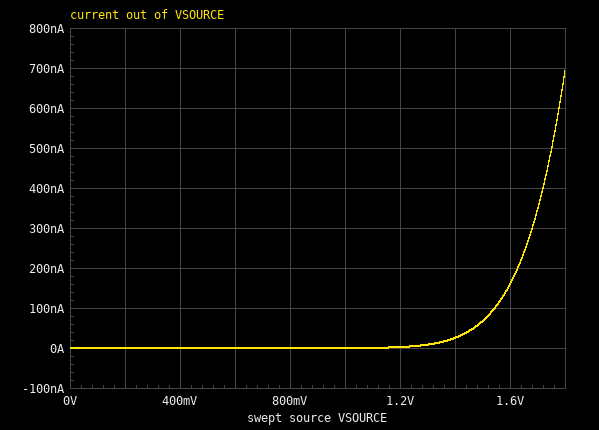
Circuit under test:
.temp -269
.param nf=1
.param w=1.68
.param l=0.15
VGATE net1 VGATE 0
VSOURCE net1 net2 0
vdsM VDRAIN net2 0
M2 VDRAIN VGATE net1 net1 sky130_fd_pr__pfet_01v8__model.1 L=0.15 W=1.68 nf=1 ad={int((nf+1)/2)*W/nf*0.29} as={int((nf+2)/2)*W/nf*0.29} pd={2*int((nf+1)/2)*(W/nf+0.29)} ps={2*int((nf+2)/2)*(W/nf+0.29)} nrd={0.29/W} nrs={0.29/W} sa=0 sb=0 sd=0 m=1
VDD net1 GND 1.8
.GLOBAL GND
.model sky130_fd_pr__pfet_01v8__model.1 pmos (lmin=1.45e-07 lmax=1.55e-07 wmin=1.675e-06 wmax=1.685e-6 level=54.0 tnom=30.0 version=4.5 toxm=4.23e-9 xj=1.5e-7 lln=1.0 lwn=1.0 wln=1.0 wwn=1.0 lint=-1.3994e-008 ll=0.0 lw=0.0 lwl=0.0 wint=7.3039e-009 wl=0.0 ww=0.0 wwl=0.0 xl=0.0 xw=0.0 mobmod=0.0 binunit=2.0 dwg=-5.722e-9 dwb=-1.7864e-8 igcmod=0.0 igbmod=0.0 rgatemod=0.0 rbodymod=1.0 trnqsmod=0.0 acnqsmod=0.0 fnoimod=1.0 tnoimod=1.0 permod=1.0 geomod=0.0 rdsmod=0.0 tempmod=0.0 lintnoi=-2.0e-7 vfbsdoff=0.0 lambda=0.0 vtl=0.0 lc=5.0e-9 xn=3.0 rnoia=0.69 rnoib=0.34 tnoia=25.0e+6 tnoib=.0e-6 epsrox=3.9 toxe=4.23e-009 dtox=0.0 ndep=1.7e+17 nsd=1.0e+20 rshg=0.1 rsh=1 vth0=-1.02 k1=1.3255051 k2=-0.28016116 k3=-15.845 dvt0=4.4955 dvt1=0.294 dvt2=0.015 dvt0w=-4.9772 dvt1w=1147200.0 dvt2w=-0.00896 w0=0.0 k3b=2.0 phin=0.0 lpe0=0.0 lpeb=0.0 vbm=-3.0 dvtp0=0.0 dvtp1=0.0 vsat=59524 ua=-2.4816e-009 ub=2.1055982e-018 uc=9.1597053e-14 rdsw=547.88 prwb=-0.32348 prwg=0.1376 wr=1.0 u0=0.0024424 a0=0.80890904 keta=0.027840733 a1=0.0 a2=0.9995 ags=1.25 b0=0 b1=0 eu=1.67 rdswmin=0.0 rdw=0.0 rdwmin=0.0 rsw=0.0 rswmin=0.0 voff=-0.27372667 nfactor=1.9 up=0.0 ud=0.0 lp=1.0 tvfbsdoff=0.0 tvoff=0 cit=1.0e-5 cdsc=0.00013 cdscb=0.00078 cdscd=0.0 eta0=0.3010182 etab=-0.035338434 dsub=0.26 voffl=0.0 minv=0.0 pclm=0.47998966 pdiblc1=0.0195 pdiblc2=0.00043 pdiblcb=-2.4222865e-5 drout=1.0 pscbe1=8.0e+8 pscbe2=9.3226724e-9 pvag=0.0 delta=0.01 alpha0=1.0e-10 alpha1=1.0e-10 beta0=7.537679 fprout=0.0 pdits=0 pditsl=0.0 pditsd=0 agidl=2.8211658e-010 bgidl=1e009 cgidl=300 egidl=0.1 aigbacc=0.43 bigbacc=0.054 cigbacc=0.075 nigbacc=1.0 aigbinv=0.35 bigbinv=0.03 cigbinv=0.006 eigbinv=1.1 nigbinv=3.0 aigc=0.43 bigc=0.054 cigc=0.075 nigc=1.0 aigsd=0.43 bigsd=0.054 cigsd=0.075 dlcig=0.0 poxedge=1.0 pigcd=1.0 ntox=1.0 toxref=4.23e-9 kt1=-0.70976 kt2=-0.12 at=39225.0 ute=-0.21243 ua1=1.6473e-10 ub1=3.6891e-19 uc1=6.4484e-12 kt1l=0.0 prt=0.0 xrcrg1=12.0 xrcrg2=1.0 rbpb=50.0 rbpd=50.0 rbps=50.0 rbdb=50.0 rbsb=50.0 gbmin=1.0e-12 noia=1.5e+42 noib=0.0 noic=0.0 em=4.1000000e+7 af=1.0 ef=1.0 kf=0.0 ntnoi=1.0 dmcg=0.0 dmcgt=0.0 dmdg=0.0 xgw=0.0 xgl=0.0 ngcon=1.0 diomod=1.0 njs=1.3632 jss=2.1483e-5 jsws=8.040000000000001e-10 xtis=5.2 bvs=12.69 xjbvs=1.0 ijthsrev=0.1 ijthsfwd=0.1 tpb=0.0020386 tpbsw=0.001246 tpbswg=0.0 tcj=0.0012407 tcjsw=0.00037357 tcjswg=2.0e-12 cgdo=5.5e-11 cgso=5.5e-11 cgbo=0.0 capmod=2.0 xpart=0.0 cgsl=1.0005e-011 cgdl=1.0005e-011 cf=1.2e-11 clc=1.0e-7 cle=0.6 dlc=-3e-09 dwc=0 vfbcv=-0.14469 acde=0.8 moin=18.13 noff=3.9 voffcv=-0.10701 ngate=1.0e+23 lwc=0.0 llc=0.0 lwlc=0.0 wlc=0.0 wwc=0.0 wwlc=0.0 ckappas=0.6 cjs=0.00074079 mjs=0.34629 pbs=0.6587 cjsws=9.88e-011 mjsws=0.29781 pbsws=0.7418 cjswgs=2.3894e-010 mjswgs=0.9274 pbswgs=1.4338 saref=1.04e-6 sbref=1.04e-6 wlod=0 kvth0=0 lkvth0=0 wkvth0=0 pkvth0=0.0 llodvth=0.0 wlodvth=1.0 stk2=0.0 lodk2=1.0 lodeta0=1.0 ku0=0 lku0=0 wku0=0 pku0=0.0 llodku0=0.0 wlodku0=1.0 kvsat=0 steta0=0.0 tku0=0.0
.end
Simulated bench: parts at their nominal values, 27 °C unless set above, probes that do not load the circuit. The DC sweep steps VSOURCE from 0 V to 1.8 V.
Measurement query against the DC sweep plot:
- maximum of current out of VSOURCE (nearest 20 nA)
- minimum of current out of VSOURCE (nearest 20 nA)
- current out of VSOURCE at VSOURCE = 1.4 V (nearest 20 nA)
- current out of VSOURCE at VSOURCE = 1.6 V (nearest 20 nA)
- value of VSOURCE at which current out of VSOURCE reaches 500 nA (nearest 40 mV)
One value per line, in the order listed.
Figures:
700 nA
0 A
20 nA
160 nA
1.76 V
